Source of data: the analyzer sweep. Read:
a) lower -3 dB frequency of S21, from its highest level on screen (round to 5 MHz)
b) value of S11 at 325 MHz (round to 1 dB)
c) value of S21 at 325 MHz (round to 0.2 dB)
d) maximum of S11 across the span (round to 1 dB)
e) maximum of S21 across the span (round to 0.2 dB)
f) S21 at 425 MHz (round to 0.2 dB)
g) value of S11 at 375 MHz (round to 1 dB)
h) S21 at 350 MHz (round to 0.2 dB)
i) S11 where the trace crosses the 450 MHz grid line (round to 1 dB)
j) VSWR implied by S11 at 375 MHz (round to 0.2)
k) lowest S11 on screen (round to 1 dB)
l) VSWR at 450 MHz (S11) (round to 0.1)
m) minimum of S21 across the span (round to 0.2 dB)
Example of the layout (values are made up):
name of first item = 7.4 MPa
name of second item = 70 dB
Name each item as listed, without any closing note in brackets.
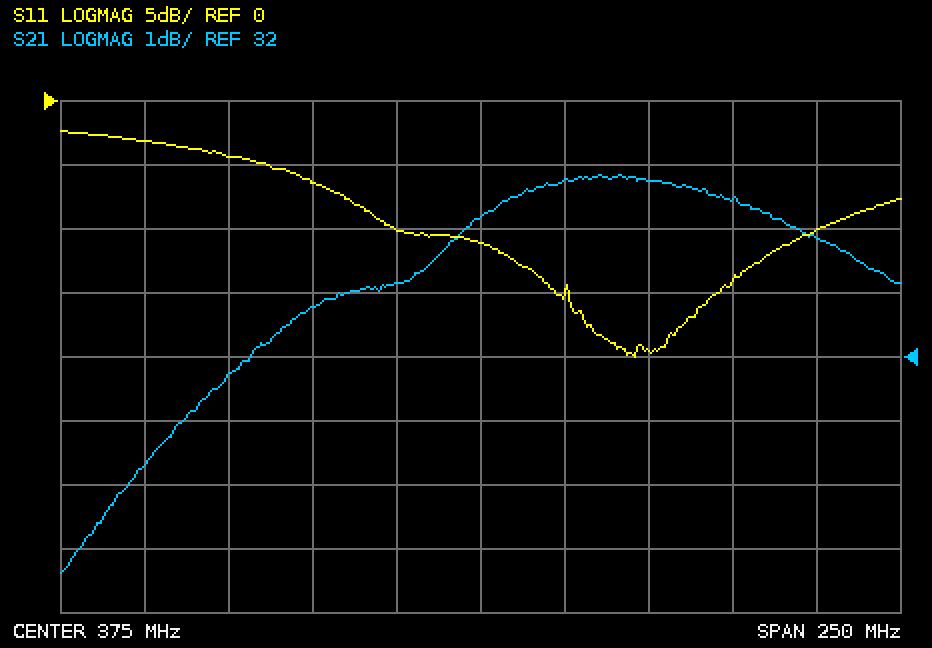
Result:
lower -3 dB frequency of S21, from its highest level on screen = 305 MHz
value of S11 at 325 MHz = -6 dB
value of S21 at 325 MHz = 32.8 dB
maximum of S11 across the span = -2 dB
maximum of S21 across the span = 34.8 dB
S21 at 425 MHz = 34.8 dB
value of S11 at 375 MHz = -11 dB
S21 at 350 MHz = 33.2 dB
S11 where the trace crosses the 450 MHz grid line = -14 dB
VSWR implied by S11 at 375 MHz = 1.8
lowest S11 on screen = -20 dB
VSWR at 450 MHz (S11) = 1.5
minimum of S21 across the span = 28.6 dB
